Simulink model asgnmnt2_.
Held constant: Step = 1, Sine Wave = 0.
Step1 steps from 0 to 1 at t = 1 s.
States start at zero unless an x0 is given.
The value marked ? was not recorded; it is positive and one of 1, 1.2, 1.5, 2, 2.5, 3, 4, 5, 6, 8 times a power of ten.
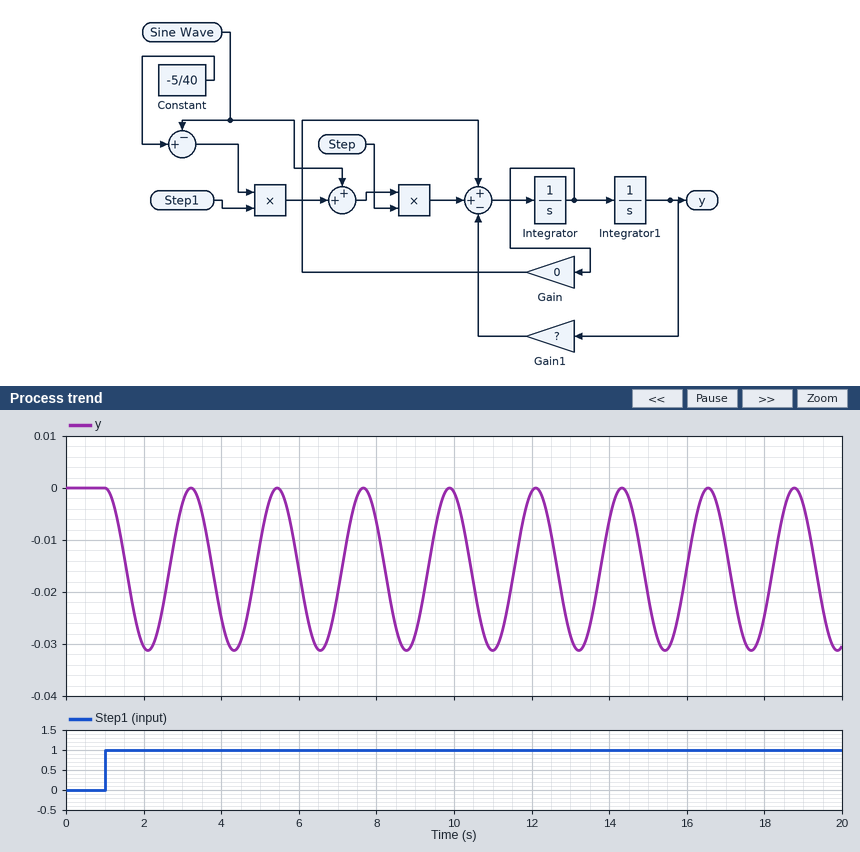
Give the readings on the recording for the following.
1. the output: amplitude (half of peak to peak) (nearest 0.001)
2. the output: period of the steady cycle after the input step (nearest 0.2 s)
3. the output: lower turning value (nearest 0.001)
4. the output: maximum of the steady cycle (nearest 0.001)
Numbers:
0.016
2.2 s
-0.031
0.000
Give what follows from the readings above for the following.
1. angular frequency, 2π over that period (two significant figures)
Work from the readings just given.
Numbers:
2.9 rad/s
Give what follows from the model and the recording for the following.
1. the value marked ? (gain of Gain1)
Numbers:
8
